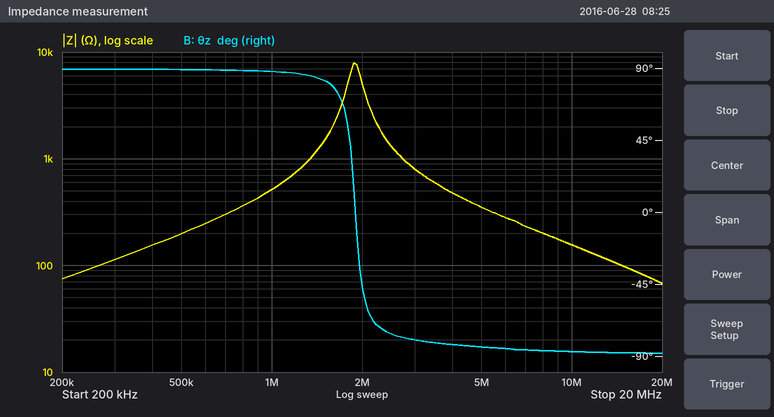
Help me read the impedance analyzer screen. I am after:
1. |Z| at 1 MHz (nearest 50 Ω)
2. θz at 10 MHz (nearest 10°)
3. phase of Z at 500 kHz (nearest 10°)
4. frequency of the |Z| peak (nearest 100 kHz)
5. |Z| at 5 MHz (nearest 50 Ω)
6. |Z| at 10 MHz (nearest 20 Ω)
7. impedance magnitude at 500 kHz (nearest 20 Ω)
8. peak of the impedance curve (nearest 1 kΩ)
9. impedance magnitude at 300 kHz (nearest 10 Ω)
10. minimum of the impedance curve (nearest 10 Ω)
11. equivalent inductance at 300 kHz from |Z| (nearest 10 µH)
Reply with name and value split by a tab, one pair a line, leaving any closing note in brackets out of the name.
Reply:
|Z| at 1 MHz	500 Ω
θz at 10 MHz	-90°
phase of Z at 500 kHz	90°
frequency of the |Z| peak	1.9 MHz
|Z| at 5 MHz	350 Ω
|Z| at 10 MHz	160 Ω
impedance magnitude at 500 kHz	200 Ω
peak of the impedance curve	8 kΩ
impedance magnitude at 300 kHz	110 Ω
minimum of the impedance curve	70 Ω
equivalent inductance at 300 kHz from |Z|	60 µH
